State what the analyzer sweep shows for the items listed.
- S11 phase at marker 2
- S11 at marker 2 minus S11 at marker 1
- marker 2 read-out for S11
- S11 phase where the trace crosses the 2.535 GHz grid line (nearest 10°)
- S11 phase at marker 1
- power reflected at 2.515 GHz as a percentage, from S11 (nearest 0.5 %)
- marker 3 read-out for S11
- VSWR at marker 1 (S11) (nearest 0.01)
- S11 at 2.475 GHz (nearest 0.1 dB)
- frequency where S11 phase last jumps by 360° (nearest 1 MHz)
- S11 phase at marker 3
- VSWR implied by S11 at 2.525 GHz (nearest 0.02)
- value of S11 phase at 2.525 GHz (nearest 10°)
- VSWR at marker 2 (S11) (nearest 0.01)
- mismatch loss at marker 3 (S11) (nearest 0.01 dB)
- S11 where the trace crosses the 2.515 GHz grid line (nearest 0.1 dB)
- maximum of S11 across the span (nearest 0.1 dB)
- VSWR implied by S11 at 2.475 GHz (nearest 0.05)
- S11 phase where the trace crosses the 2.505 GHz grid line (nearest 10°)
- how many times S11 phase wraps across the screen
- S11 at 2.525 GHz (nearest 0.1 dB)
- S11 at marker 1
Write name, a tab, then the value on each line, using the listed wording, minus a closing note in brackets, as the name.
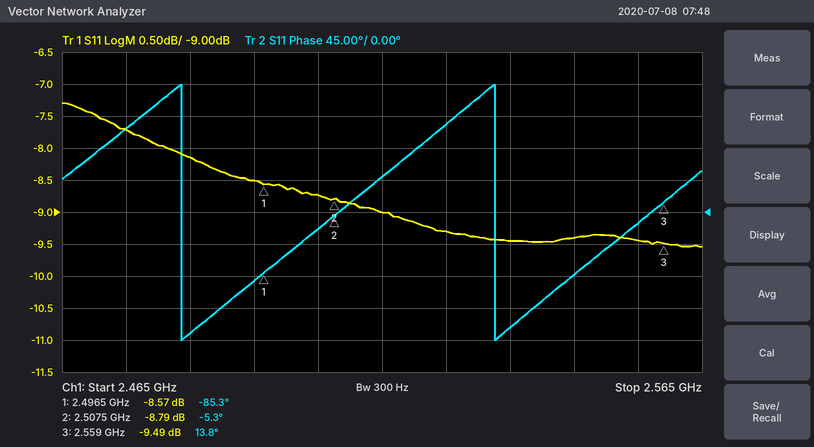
S11 phase at marker 2	-5.3°
S11 at marker 2 minus S11 at marker 1	-0.22 dB
marker 2 read-out for S11	-8.79 dB
S11 phase where the trace crosses the 2.535 GHz grid line	-160°
S11 phase at marker 1	-85.3°
power reflected at 2.515 GHz as a percentage, from S11	12.5 %
marker 3 read-out for S11	-9.49 dB
VSWR at marker 1 (S11)	2.19
S11 at 2.475 GHz	-7.7 dB
frequency where S11 phase last jumps by 360°	2.533 GHz
S11 phase at marker 3	13.8°
VSWR implied by S11 at 2.525 GHz	2.04
value of S11 phase at 2.525 GHz	120°
VSWR at marker 2 (S11)	2.14
mismatch loss at marker 3 (S11)	0.52 dB
S11 where the trace crosses the 2.515 GHz grid line	-9.0 dB
maximum of S11 across the span	-7.3 dB
VSWR implied by S11 at 2.475 GHz	2.40
S11 phase where the trace crosses the 2.505 GHz grid line	-20°
how many times S11 phase wraps across the screen	2
S11 at 2.525 GHz	-9.3 dB
S11 at marker 1	-8.57 dB
